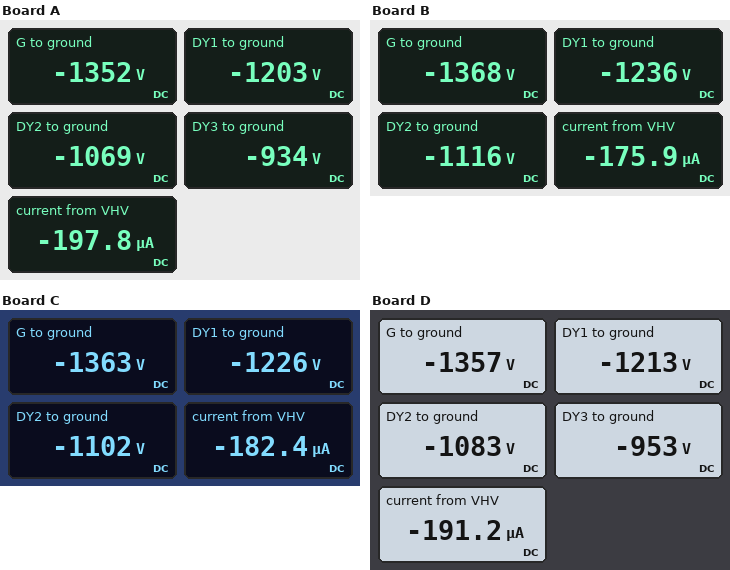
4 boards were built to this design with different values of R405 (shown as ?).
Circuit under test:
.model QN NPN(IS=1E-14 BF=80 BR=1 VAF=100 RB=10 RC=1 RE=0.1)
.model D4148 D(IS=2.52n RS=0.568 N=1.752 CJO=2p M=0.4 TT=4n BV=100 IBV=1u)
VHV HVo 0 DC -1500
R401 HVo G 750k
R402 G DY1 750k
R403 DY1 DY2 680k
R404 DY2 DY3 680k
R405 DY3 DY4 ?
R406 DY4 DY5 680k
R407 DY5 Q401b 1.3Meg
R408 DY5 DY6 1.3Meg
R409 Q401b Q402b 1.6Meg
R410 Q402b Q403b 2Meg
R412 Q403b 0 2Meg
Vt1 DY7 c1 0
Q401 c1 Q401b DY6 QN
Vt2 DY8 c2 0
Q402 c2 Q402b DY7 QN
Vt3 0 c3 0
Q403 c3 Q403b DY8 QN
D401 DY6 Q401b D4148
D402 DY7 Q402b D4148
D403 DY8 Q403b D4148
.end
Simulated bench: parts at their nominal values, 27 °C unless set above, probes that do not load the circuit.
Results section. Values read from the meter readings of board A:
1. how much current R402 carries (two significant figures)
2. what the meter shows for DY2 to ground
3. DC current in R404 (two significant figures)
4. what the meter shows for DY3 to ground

200 µA
-1069 V
200 µA
-934 V
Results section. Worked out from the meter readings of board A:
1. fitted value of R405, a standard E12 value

560 kΩ
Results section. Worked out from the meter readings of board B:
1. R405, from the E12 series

1.5 MΩ
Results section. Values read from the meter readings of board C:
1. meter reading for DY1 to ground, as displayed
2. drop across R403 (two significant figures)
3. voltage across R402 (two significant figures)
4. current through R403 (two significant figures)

-1226 V
120 V
140 V
180 µA
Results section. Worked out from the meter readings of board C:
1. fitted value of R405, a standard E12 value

1.2 MΩ
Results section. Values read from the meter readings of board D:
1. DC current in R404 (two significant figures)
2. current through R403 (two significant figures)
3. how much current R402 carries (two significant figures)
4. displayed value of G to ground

190 µA
190 µA
190 µA
-1357 V
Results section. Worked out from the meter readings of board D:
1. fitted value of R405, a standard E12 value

820 kΩ
